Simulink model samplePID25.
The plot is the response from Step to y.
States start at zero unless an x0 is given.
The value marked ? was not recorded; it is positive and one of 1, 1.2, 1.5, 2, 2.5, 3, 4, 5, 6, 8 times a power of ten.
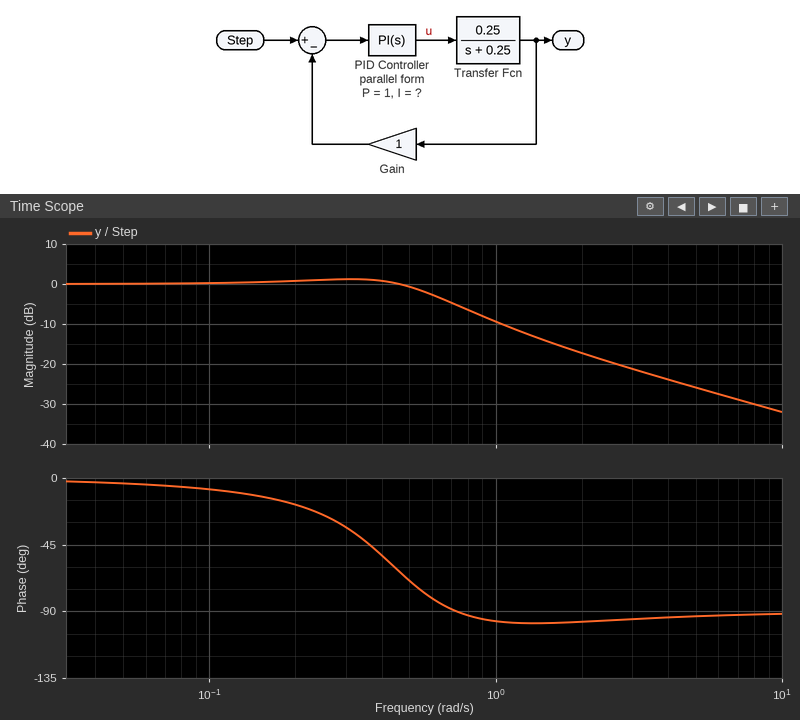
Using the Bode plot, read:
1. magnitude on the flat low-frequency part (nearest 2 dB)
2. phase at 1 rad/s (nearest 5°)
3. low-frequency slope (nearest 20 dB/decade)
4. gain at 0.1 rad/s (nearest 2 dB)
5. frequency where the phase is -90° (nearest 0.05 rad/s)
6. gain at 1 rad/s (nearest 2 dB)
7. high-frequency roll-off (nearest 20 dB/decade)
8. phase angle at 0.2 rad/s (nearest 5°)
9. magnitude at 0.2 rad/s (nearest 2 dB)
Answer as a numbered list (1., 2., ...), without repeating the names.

1. 0 dB
2. -95°
3. 0 dB/decade
4. 0 dB
5. 0.75 rad/s
6. -10 dB
7. -20 dB/decade
8. -20°
9. 0 dB
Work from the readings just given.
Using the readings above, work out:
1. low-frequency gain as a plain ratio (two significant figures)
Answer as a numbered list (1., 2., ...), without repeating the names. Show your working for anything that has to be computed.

1. 10^(0 / 20) = 1.0
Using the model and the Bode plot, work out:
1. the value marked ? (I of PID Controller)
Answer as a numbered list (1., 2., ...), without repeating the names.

1. 0.8
